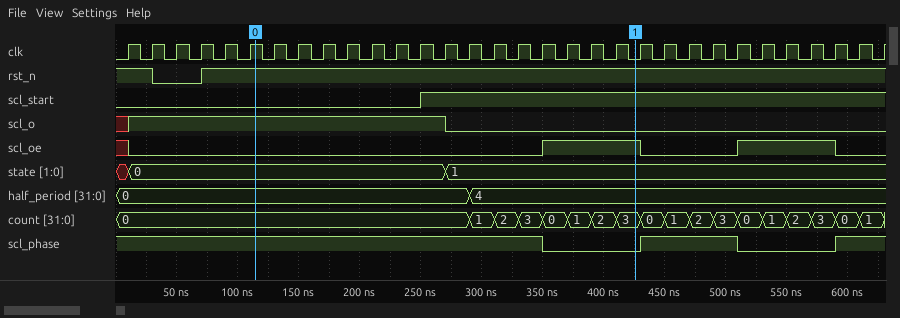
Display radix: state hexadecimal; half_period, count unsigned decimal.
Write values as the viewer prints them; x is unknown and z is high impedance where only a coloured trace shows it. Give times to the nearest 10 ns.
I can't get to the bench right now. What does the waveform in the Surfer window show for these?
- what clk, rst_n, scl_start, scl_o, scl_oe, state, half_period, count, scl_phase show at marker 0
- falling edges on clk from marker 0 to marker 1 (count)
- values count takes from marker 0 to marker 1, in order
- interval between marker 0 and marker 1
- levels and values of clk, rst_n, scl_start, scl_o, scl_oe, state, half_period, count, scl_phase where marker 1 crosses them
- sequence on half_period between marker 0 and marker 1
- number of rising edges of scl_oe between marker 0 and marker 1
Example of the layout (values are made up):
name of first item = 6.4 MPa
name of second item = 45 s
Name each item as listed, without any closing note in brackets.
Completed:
what clk, rst_n, scl_start, scl_o, scl_oe, state, half_period, count, scl_phase show at marker 0 = clk=1, rst_n=1, scl_start=0, scl_o=1, scl_oe=0, state=0, half_period=0, count=0, scl_phase=1
falling edges on clk from marker 0 to marker 1 = 16
values count takes from marker 0 to marker 1, in order = 0, 1, 2, 3, 0, 1, 2, 3
interval between marker 0 and marker 1 = 310 ns
levels and values of clk, rst_n, scl_start, scl_o, scl_oe, state, half_period, count, scl_phase where marker 1 crosses them = clk=0, rst_n=1, scl_start=1, scl_o=0, scl_oe=1, state=1, half_period=4, count=3, scl_phase=0
sequence on half_period between marker 0 and marker 1 = 0, 4
number of rising edges of scl_oe between marker 0 and marker 1 = 1
